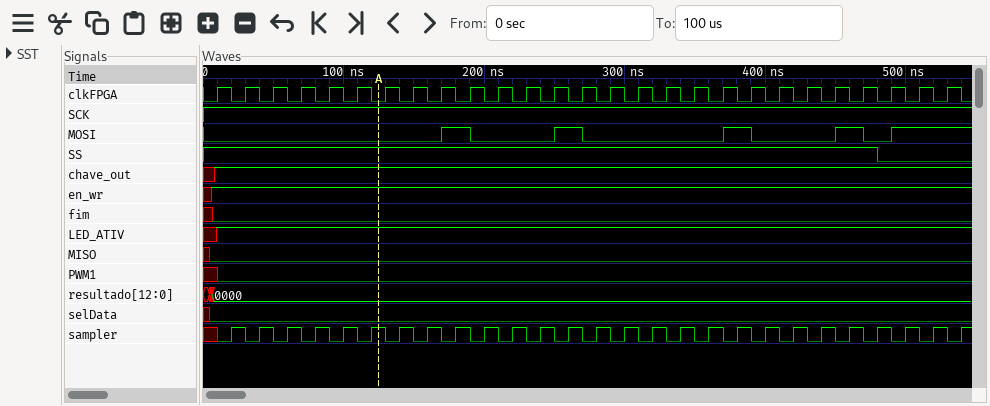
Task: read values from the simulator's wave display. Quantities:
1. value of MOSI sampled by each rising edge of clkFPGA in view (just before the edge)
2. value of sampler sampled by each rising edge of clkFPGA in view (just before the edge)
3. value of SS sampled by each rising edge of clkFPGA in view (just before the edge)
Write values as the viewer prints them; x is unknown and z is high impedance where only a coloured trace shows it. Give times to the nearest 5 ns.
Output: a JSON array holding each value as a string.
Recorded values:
["0 0 0 0 0 0 0 0 0 1 0 0 0 1 0 0 0 0 0 1 0 0 0 1 0 1 1", "x 1 1 1 1 1 1 1 1 1 1 1 1 1 1 1 1 1 1 1 1 1 1 1 1 1 1", "1 1 1 1 1 1 1 1 1 1 1 1 1 1 1 1 1 1 1 1 1 1 1 1 0 0 0"]
